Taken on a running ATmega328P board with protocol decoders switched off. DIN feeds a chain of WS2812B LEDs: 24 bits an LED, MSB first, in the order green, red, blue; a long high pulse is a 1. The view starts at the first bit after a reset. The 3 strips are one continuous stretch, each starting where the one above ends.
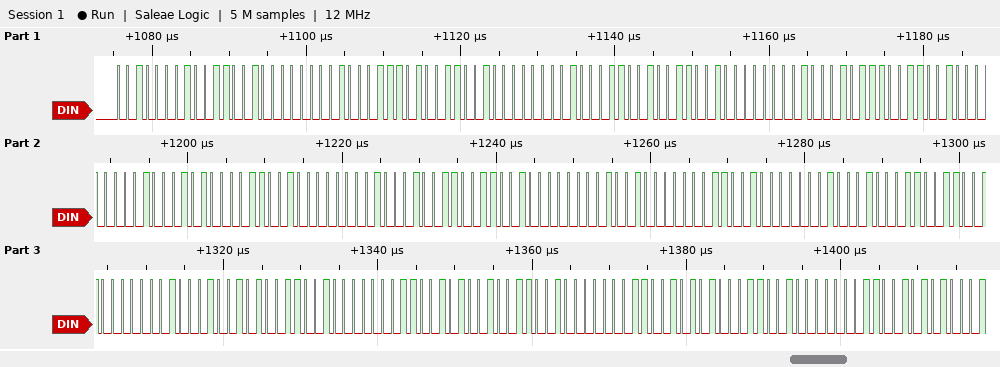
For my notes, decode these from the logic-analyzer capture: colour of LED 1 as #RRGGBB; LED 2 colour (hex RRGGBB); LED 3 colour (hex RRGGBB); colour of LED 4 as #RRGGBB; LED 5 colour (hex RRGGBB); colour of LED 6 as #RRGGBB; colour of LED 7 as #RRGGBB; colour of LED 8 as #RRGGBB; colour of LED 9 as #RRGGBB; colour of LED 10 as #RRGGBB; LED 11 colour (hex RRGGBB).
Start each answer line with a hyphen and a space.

- #322101
- #321D01
- #321901
- #321701
- #321401
- #321301
- #322002
- #322302
- #322503
- #322903
- #322A03
